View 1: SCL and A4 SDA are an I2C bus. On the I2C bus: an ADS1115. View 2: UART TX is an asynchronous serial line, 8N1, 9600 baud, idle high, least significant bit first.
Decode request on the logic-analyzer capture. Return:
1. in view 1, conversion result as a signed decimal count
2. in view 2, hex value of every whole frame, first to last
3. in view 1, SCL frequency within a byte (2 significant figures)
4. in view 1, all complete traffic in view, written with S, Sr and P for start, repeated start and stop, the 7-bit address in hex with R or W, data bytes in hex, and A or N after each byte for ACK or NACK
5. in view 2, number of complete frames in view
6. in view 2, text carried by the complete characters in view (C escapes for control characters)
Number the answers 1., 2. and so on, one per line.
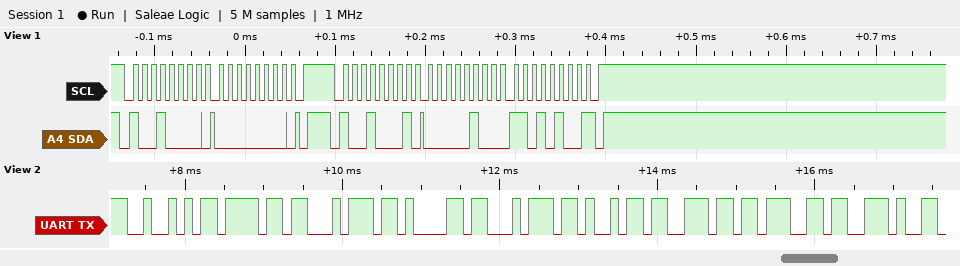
1. 1236
2. 0x52 0x6F 0x74 0x61 0x74 0x69 0x6E 0x67 0x2E
3. 100 kHz
4. S 48W A 00 A P S 48R A 04 A D4 N P
5. 9
6. "Rotating."
